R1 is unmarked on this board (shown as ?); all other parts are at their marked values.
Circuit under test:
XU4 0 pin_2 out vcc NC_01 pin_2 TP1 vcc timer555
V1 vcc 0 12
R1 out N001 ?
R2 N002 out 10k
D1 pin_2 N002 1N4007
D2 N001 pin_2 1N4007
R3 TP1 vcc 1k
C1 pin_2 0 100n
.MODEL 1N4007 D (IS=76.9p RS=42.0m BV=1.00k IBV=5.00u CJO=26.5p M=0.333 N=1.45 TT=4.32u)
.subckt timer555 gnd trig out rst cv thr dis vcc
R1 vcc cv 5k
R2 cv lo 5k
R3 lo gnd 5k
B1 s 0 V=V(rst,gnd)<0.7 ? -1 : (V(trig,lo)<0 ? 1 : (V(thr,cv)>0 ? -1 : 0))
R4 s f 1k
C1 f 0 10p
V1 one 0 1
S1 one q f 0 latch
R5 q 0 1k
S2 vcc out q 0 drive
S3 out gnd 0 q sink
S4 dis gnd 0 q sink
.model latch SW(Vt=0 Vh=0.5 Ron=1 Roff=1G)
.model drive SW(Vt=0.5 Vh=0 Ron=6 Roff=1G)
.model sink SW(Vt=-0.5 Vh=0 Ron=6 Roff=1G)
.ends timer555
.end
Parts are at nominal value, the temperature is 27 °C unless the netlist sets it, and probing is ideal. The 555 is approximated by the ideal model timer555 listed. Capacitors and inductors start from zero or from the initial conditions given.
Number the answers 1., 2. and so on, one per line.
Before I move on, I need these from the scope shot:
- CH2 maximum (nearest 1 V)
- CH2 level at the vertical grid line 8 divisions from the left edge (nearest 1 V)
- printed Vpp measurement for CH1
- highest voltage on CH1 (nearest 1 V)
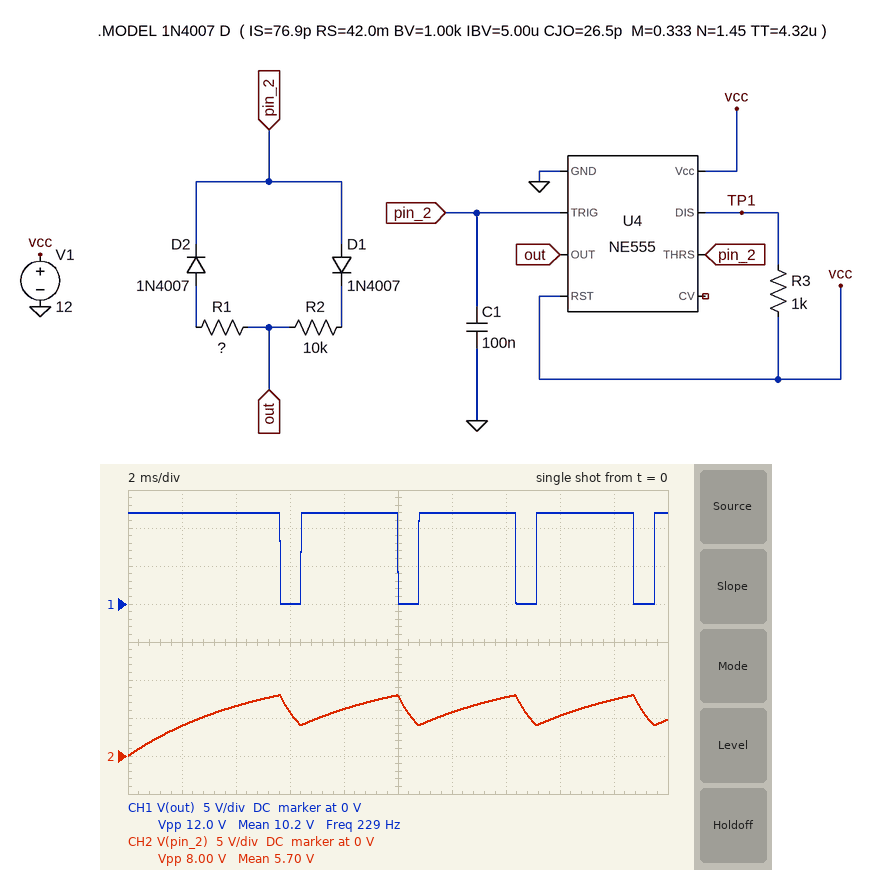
1. 8 V
2. 5 V
3. 12.0 V
4. 12 V
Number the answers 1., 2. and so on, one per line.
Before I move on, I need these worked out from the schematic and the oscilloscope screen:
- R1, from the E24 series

1. 47 kΩ
